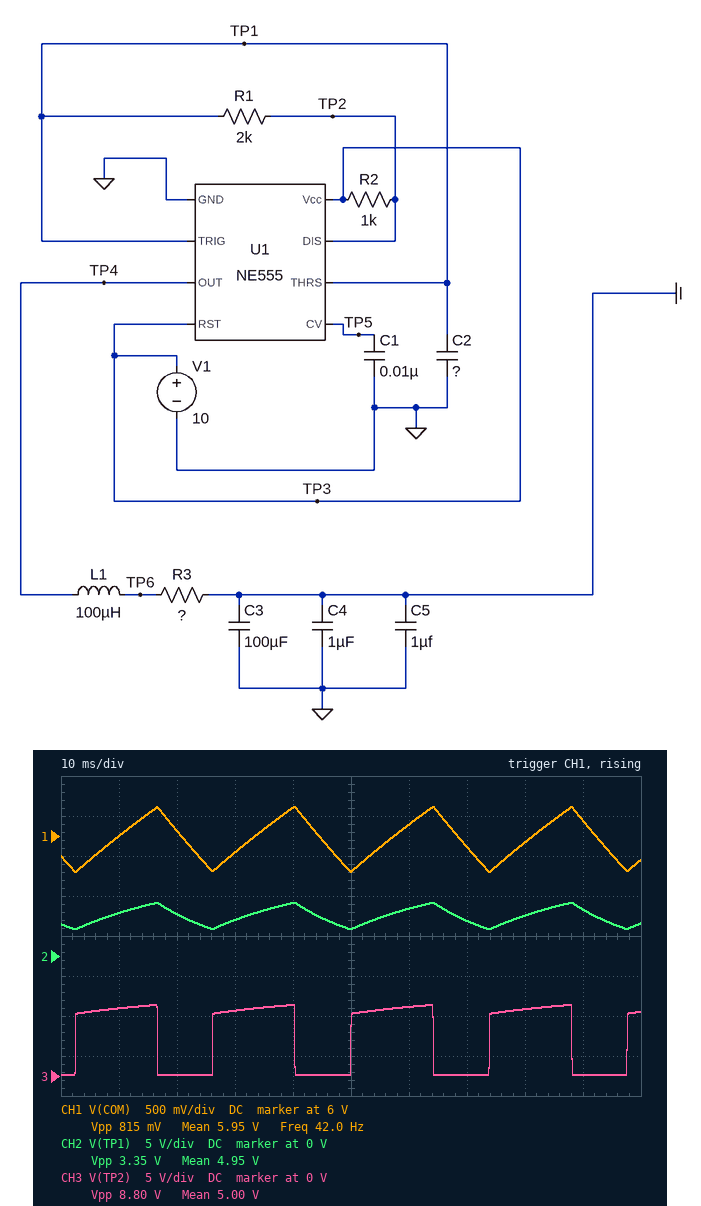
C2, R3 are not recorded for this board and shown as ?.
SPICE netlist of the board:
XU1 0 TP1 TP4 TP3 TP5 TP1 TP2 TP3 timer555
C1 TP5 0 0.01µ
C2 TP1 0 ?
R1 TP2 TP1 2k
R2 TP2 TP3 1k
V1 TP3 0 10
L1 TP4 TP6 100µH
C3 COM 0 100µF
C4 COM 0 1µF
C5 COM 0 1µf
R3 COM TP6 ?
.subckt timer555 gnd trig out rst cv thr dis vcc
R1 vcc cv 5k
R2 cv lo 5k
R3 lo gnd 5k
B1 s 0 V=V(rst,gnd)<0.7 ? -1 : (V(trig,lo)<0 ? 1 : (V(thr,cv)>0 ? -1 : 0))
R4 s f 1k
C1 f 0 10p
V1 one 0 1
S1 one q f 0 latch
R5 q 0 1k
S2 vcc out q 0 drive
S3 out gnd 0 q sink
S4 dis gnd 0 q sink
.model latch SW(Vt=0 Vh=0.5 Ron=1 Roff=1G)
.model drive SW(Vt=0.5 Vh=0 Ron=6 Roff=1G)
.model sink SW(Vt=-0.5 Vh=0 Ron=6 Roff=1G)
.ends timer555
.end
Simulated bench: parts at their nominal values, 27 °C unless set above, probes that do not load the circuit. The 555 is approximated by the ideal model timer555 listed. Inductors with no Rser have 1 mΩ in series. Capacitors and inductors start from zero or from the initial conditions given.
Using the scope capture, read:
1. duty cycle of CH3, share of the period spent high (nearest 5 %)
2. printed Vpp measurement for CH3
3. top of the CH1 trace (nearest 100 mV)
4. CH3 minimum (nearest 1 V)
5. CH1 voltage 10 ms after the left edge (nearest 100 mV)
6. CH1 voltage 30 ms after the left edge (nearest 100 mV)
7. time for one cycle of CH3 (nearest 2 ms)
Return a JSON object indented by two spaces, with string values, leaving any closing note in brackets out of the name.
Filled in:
{
  "duty cycle of CH3, share of the period spent high": "60 %",
  "printed Vpp measurement for CH3": "8.80 V",
  "top of the CH1 trace": "6.4 V",
  "CH3 minimum": "0 V",
  "CH1 voltage 10 ms after the left edge": "6.0 V",
  "CH1 voltage 30 ms after the left edge": "5.8 V",
  "time for one cycle of CH3": "24 ms"
}
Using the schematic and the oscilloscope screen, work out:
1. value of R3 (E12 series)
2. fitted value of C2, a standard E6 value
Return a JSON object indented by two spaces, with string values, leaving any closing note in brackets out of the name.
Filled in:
{
  "value of R3": "680 Ω",
  "fitted value of C2, a standard E6 value": "6.8 µF"
}
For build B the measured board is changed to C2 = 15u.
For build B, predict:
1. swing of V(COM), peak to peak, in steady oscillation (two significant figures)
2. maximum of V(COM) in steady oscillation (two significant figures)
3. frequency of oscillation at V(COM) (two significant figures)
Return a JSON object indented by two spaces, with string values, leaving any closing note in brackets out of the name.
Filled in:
{
  "swing of V(COM), peak to peak, in steady oscillation": "1.8 V",
  "maximum of V(COM) in steady oscillation": "6.8 V",
  "frequency of oscillation at V(COM)": "19 Hz"
}
